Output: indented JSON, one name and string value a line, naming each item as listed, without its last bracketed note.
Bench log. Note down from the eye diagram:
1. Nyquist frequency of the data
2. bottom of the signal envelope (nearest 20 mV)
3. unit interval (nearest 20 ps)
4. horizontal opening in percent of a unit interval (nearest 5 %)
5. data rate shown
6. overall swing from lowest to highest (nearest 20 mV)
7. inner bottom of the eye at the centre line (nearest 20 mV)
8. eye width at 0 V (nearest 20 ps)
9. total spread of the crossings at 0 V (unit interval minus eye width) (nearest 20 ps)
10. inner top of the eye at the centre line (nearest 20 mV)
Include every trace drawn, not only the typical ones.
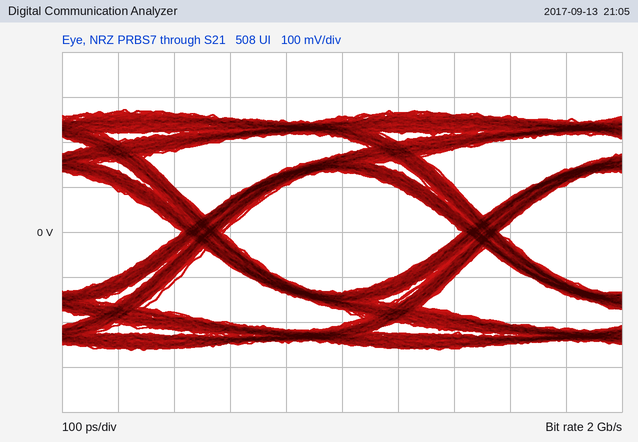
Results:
{
  "Nyquist frequency of the data": "1 GHz",
  "bottom of the signal envelope": "-260 mV",
  "unit interval": "500 ps",
  "horizontal opening in percent of a unit interval": "85 %",
  "data rate shown": "2 Gb/s",
  "overall swing from lowest to highest": "540 mV",
  "inner bottom of the eye at the centre line": "-140 mV",
  "eye width at 0 V": "420 ps",
  "total spread of the crossings at 0 V (unit interval minus eye width)": "80 ps",
  "inner top of the eye at the centre line": "140 mV"
}
